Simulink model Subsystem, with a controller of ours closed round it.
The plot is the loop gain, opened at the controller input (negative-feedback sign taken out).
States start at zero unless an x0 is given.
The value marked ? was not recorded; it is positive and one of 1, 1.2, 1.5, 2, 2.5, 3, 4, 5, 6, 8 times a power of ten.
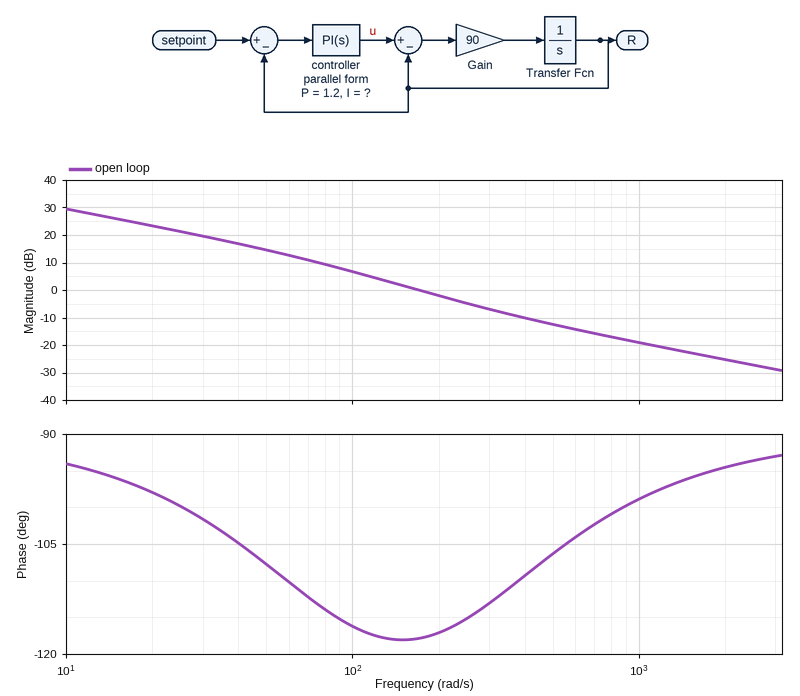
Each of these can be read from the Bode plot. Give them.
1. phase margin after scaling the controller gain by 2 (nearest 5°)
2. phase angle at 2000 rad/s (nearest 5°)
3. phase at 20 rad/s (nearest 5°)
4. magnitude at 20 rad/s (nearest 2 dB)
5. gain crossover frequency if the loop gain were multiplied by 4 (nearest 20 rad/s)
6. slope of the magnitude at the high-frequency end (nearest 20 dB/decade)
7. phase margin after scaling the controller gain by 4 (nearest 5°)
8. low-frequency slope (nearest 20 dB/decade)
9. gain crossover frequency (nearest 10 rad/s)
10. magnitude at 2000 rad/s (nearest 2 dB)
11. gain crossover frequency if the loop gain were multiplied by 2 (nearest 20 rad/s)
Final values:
65°
-95°
-100°
24 dB
480 rad/s
-20 dB/decade
75°
-20 dB/decade
170 rad/s
-26 dB
280 rad/s
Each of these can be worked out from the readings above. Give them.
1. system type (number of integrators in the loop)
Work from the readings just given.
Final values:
1
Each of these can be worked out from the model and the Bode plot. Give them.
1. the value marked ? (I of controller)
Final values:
300
